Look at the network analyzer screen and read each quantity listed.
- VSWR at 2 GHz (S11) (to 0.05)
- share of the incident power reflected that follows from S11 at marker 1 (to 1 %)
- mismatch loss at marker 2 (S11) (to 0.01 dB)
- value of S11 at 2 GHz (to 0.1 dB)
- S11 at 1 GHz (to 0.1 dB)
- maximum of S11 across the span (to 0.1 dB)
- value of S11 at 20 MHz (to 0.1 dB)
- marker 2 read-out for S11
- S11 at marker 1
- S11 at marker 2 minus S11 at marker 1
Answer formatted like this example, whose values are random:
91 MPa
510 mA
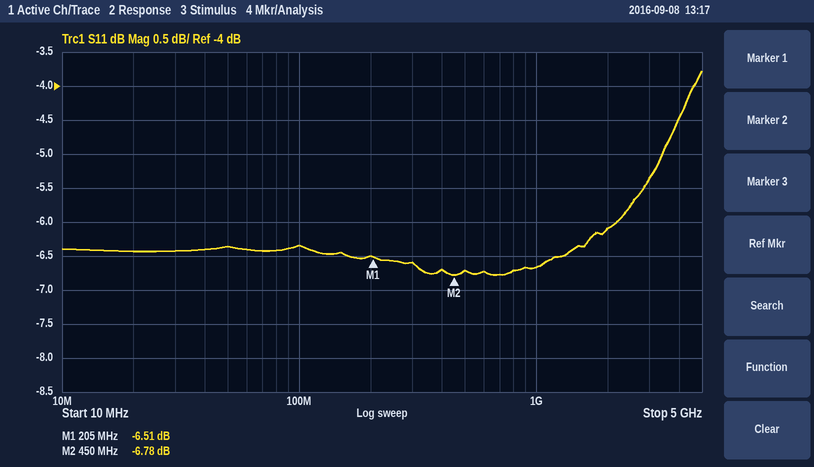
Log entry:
2.95
22 %
1.02 dB
-6.1 dB
-6.7 dB
-3.8 dB
-6.4 dB
-6.78 dB
-6.51 dB
-0.27 dB
